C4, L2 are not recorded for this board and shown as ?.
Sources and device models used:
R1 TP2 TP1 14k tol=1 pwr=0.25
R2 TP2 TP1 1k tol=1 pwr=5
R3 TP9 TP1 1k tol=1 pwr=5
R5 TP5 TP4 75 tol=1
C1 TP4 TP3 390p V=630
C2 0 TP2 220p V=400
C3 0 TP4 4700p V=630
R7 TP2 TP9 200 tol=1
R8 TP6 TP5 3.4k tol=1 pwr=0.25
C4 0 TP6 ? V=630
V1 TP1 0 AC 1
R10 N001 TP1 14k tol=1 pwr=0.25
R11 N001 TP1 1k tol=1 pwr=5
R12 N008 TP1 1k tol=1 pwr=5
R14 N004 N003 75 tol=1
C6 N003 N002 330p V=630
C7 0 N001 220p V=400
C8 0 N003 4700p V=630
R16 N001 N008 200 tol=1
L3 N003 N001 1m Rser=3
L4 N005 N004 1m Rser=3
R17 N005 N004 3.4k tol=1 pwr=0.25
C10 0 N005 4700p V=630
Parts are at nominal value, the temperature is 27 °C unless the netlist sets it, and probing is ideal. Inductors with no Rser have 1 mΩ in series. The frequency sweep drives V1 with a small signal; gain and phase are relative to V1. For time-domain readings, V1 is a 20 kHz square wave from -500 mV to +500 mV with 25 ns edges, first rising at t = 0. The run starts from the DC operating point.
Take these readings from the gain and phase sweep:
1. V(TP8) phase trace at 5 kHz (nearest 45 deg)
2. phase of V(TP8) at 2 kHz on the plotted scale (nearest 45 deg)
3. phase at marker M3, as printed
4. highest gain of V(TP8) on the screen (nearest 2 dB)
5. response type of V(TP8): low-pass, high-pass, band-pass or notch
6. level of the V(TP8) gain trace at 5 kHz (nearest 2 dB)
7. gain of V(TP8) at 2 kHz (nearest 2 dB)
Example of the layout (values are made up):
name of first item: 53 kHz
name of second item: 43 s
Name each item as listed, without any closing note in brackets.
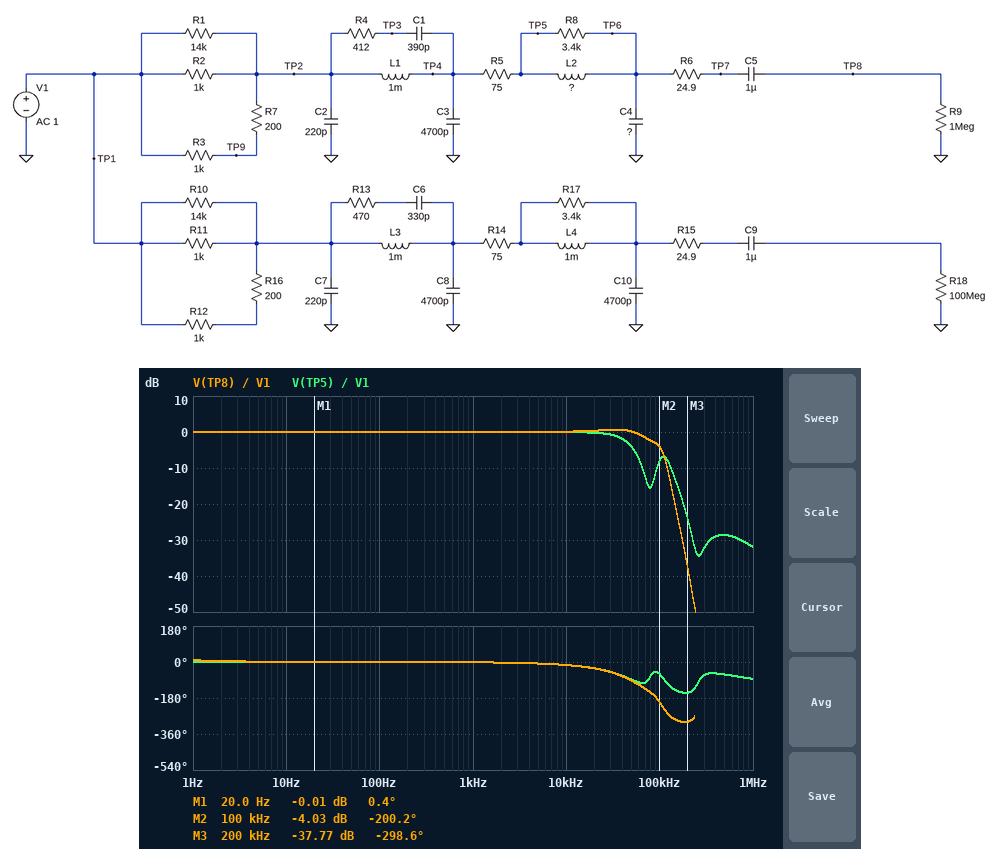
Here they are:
V(TP8) phase trace at 5 kHz: 0 deg
phase of V(TP8) at 2 kHz on the plotted scale: 0 deg
phase at marker M3, as printed: -298.6 deg
highest gain of V(TP8) on the screen: 0 dB
response type of V(TP8): low-pass, high-pass, band-pass or notch: low-pass
level of the V(TP8) gain trace at 5 kHz: 0 dB
gain of V(TP8) at 2 kHz: 0 dB
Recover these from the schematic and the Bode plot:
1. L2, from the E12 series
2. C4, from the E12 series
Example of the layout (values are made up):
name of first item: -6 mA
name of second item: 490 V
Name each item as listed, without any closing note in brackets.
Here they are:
L2, from the E12 series: 1.5 mH
C4, from the E12 series: 2.7 nF
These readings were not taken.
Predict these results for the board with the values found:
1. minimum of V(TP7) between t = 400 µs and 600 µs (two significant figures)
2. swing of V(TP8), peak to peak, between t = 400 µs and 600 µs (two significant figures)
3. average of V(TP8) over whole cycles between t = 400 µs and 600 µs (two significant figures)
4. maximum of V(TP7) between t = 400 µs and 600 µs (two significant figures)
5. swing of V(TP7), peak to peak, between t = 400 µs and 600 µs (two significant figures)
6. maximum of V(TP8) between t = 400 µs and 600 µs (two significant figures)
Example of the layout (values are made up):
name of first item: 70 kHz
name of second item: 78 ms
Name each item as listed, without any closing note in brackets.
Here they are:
minimum of V(TP7) between t = 400 µs and 600 µs: -640 mV
swing of V(TP8), peak to peak, between t = 400 µs and 600 µs: 1.3 V
average of V(TP8) over whole cycles between t = 400 µs and 600 µs: 500 mV
maximum of V(TP7) between t = 400 µs and 600 µs: 640 mV
swing of V(TP7), peak to peak, between t = 400 µs and 600 µs: 1.3 V
maximum of V(TP8) between t = 400 µs and 600 µs: 1.1 V
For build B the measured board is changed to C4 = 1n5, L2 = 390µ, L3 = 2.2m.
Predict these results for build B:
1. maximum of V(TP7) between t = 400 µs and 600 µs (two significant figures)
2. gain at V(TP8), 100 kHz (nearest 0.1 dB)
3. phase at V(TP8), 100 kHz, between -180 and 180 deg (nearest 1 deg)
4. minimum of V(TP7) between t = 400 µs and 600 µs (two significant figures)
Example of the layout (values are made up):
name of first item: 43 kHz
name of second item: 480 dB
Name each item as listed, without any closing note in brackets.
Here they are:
maximum of V(TP7) between t = 400 µs and 600 µs: 570 mV
gain at V(TP8), 100 kHz: -7.3 dB
phase at V(TP8), 100 kHz, between -180 and 180 deg: -139 deg
minimum of V(TP7) between t = 400 µs and 600 µs: -570 mV
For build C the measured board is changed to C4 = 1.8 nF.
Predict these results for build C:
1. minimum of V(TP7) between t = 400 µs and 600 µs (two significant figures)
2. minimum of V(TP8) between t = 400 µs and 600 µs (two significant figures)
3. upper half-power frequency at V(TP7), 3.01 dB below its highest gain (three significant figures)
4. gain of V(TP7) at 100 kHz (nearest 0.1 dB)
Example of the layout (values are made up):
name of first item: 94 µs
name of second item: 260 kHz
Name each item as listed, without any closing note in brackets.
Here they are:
minimum of V(TP7) between t = 400 µs and 600 µs: -660 mV
minimum of V(TP8) between t = 400 µs and 600 µs: -160 mV
upper half-power frequency at V(TP7), 3.01 dB below its highest gain: 88.8 kHz
gain of V(TP7) at 100 kHz: -2.9 dB
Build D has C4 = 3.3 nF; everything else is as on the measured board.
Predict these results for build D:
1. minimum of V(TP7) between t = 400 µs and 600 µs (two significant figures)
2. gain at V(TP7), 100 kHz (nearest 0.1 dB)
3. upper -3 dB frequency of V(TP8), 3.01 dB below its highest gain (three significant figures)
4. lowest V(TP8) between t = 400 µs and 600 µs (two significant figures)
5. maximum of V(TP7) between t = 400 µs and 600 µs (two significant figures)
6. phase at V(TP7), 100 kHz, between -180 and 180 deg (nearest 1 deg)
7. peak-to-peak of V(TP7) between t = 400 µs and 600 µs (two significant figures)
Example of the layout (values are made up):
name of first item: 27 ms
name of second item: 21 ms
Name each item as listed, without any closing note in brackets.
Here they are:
minimum of V(TP7) between t = 400 µs and 600 µs: -620 mV
gain at V(TP7), 100 kHz: -5.4 dB
upper -3 dB frequency of V(TP8), 3.01 dB below its highest gain: 72.8 kHz
lowest V(TP8) between t = 400 µs and 600 µs: -120 mV
maximum of V(TP7) between t = 400 µs and 600 µs: 620 mV
phase at V(TP7), 100 kHz, between -180 and 180 deg: 147 deg
peak-to-peak of V(TP7) between t = 400 µs and 600 µs: 1.2 V
